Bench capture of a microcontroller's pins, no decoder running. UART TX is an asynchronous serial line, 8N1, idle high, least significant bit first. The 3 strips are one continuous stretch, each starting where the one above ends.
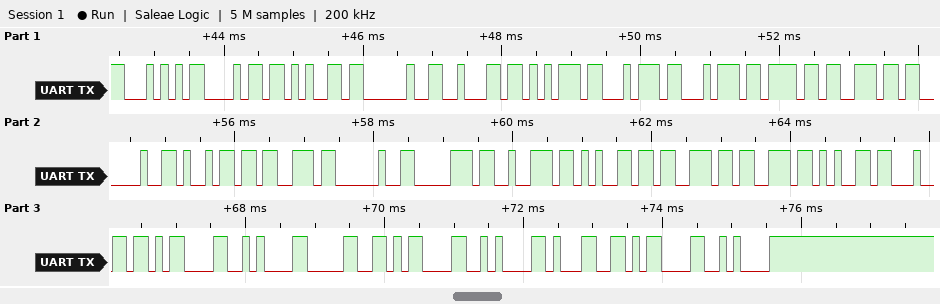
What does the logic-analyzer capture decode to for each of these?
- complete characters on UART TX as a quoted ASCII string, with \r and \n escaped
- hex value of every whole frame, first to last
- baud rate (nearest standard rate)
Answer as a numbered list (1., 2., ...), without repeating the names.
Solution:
1. "The button is pressed\r\n0\r\n1\r\n"
2. 0x54 0x68 0x65 0x20 0x62 0x75 0x74 0x74 0x6F 0x6E 0x20 0x69 0x73 0x20 0x70 0x72 0x65 0x73 0x73 0x65 0x64 0x0D 0x0A 0x30 0x0D 0x0A 0x31 0x0D 0x0A
3. 9600 baud
